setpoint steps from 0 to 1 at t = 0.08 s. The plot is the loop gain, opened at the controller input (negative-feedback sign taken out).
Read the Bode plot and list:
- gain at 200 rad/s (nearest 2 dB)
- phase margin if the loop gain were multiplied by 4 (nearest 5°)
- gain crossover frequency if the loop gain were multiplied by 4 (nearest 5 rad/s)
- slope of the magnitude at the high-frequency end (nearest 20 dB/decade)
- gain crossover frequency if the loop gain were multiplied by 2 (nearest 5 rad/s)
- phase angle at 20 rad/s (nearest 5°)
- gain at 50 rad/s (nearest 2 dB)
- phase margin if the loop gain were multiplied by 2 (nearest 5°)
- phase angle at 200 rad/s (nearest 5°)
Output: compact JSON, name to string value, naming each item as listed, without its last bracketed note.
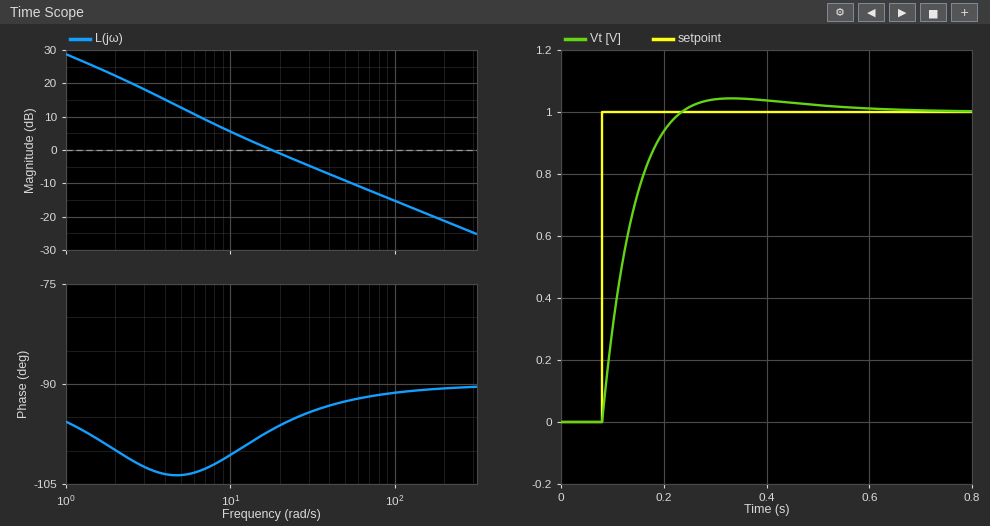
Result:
{"gain at 200 rad/s": "-22 dB", "phase margin if the loop gain were multiplied by 4": "90°", "gain crossover frequency if the loop gain were multiplied by 4": "70 rad/s", "slope of the magnitude at the high-frequency end": "-20 dB/decade", "gain crossover frequency if the loop gain were multiplied by 2": "35 rad/s", "phase angle at 20 rad/s": "-95°", "gain at 50 rad/s": "-10 dB", "phase margin if the loop gain were multiplied by 2": "85°", "phase angle at 200 rad/s": "-90°"}
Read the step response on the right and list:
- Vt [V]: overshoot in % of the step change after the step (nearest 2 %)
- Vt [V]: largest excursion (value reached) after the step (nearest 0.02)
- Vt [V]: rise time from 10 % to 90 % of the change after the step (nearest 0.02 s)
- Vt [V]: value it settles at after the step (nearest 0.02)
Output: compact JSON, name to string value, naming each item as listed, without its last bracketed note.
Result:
{"Vt [V]: overshoot in % of the step change after the step": "4 %", "Vt [V]: largest excursion (value reached) after the step": "1.04", "Vt [V]: rise time from 10 % to 90 % of the change after the step": "0.10 s", "Vt [V]: value it settles at after the step": "1.00"}
